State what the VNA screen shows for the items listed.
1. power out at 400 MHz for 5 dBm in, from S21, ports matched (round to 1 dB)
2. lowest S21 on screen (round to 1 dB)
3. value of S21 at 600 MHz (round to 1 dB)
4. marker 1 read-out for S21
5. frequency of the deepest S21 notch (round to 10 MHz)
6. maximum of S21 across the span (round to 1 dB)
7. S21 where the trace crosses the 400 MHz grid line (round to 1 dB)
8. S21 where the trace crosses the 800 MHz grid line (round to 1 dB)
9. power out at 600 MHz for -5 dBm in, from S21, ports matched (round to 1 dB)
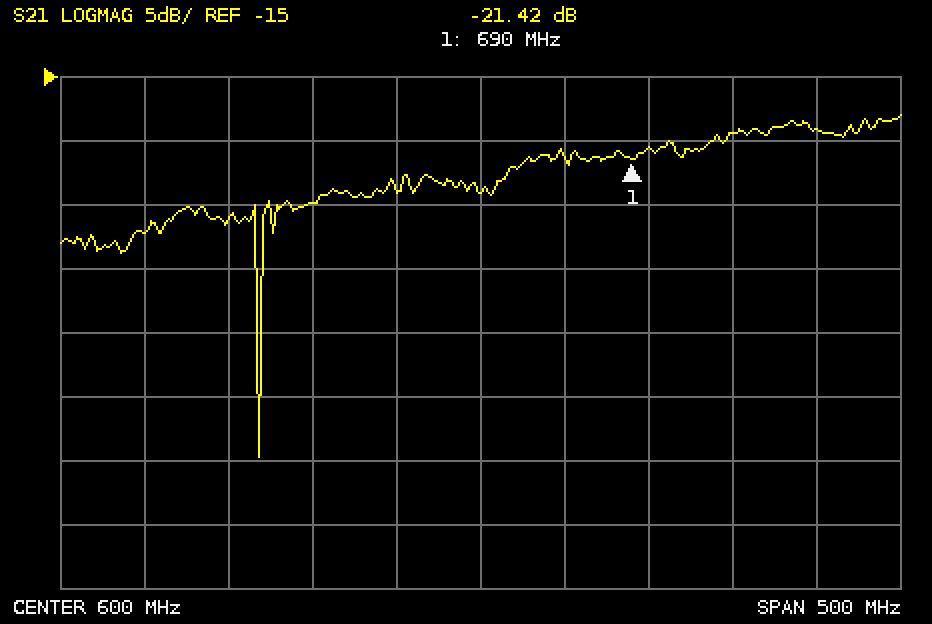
-22 dBm
-45 dB
-24 dB
-21.42 dB
470 MHz
-18 dB
-27 dB
-19 dB
-29 dBm
